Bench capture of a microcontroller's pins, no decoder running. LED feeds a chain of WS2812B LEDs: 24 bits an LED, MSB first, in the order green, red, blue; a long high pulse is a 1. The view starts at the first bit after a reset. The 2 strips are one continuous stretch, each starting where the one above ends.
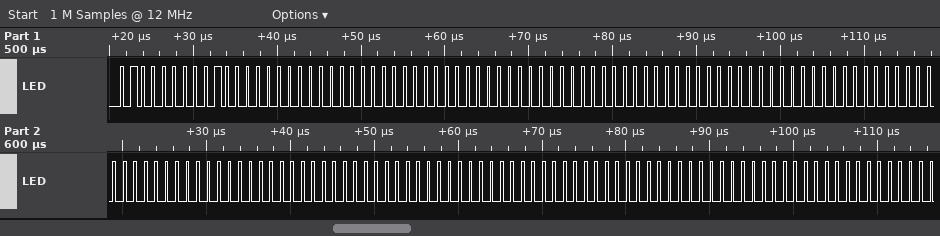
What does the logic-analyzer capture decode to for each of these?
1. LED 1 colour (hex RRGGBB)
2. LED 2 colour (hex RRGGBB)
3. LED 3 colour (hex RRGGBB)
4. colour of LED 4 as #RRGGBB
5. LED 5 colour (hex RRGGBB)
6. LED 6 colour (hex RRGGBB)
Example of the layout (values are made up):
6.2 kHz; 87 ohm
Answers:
#404000; #000000; #000000; #000000; #000000; #000000
